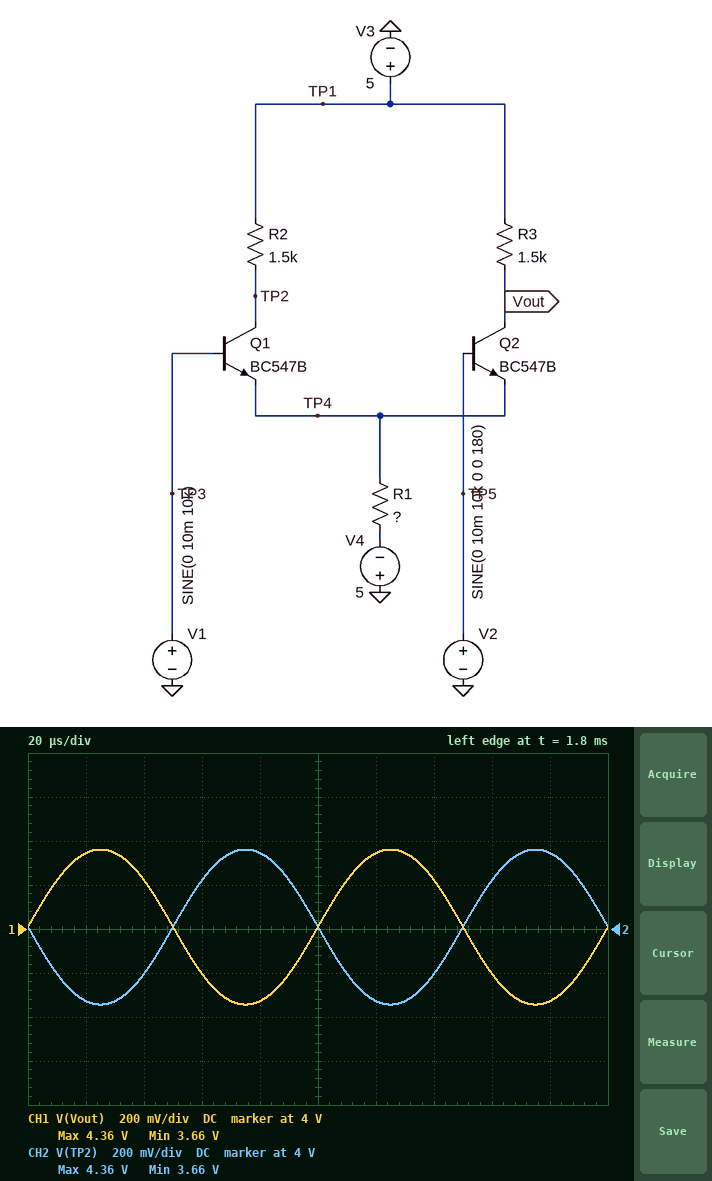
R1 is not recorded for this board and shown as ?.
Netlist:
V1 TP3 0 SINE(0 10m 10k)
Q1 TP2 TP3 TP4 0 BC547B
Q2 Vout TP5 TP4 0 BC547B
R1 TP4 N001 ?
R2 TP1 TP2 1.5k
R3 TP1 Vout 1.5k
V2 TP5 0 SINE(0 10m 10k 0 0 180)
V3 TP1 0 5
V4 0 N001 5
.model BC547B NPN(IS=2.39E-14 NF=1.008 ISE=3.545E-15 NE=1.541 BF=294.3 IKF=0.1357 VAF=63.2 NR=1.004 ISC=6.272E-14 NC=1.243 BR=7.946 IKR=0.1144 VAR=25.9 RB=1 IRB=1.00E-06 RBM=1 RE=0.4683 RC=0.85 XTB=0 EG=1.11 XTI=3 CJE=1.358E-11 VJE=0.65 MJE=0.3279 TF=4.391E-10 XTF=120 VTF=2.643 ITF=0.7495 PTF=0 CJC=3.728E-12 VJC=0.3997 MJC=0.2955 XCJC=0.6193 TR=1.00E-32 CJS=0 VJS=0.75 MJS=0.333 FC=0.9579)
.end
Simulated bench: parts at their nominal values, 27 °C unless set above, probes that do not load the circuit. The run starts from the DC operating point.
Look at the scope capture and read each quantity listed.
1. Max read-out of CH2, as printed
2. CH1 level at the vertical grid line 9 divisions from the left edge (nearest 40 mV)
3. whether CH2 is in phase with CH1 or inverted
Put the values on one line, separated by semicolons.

4.36 V; 3.68 V; inverted
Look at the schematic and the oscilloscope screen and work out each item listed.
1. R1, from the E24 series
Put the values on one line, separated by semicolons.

3.3 kΩ
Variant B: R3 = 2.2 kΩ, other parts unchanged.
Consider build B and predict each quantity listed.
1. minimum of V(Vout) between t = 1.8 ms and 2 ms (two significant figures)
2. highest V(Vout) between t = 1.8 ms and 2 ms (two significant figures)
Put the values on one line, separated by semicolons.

3.0 V; 4.1 V
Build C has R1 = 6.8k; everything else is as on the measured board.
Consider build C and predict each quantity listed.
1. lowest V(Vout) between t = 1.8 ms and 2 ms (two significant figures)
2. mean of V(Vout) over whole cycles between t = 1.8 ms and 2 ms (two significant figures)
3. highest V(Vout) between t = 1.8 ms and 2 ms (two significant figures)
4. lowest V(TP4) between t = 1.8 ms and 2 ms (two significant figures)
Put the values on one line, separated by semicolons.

4.3 V; 4.5 V; 4.7 V; -610 mV
